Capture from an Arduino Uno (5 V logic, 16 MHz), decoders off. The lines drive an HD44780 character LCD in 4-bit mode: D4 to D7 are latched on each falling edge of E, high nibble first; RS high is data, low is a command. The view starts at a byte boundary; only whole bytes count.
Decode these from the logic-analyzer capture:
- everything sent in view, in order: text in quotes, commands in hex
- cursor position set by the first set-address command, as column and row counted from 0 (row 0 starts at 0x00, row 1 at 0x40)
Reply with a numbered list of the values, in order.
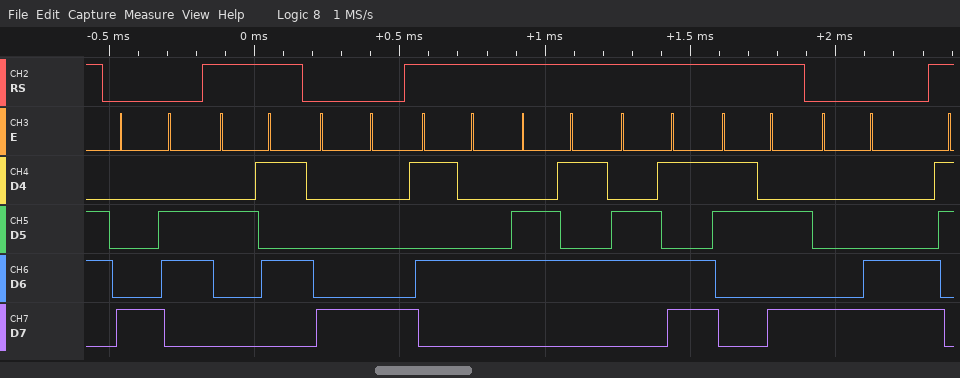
1. 0x86 "%" 0x88 "Tem:" 0x8C
2. column 6, row 0
